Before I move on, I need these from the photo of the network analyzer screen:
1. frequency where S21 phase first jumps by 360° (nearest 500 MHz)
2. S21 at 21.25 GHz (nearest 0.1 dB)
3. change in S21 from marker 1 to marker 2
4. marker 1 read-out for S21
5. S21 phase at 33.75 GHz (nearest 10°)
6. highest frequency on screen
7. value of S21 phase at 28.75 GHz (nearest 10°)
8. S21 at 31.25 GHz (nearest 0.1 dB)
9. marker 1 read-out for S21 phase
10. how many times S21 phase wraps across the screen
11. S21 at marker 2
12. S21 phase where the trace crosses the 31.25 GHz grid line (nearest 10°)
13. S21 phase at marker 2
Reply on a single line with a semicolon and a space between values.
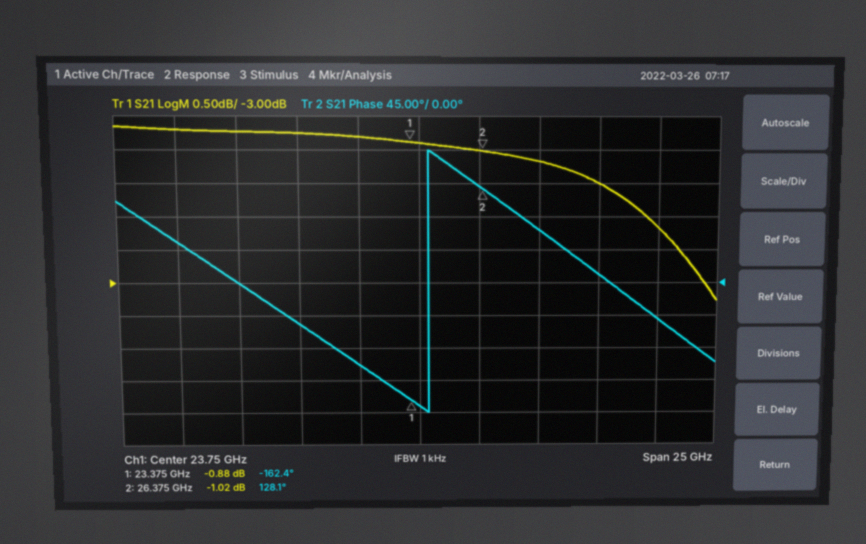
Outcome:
24.0 GHz; -0.8 dB; -0.14 dB; -0.88 dB; -50°; 36.25 GHz; 70°; -1.5 dB; -162.4°; 1; -1.02 dB; 10°; 128.1°
